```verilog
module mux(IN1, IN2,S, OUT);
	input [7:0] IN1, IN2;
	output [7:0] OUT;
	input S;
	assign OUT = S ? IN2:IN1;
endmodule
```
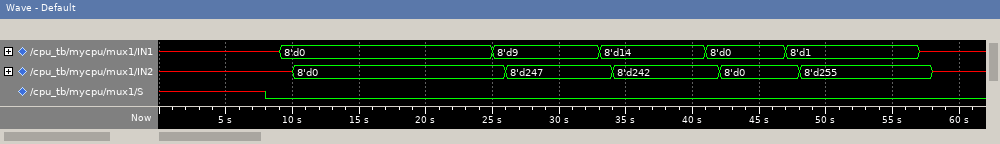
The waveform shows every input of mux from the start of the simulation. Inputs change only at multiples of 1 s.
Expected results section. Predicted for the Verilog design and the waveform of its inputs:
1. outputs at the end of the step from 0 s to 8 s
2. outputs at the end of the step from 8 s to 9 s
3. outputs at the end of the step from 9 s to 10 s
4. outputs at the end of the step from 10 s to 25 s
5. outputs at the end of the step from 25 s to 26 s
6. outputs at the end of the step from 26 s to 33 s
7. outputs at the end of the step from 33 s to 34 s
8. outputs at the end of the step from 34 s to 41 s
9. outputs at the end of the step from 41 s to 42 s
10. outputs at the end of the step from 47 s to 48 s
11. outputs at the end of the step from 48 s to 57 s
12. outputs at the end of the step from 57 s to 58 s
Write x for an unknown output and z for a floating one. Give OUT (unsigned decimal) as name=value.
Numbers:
OUT=x
OUT=x
OUT=0
OUT=0
OUT=9
OUT=9
OUT=14
OUT=14
OUT=0
OUT=1
OUT=1
OUT=x
